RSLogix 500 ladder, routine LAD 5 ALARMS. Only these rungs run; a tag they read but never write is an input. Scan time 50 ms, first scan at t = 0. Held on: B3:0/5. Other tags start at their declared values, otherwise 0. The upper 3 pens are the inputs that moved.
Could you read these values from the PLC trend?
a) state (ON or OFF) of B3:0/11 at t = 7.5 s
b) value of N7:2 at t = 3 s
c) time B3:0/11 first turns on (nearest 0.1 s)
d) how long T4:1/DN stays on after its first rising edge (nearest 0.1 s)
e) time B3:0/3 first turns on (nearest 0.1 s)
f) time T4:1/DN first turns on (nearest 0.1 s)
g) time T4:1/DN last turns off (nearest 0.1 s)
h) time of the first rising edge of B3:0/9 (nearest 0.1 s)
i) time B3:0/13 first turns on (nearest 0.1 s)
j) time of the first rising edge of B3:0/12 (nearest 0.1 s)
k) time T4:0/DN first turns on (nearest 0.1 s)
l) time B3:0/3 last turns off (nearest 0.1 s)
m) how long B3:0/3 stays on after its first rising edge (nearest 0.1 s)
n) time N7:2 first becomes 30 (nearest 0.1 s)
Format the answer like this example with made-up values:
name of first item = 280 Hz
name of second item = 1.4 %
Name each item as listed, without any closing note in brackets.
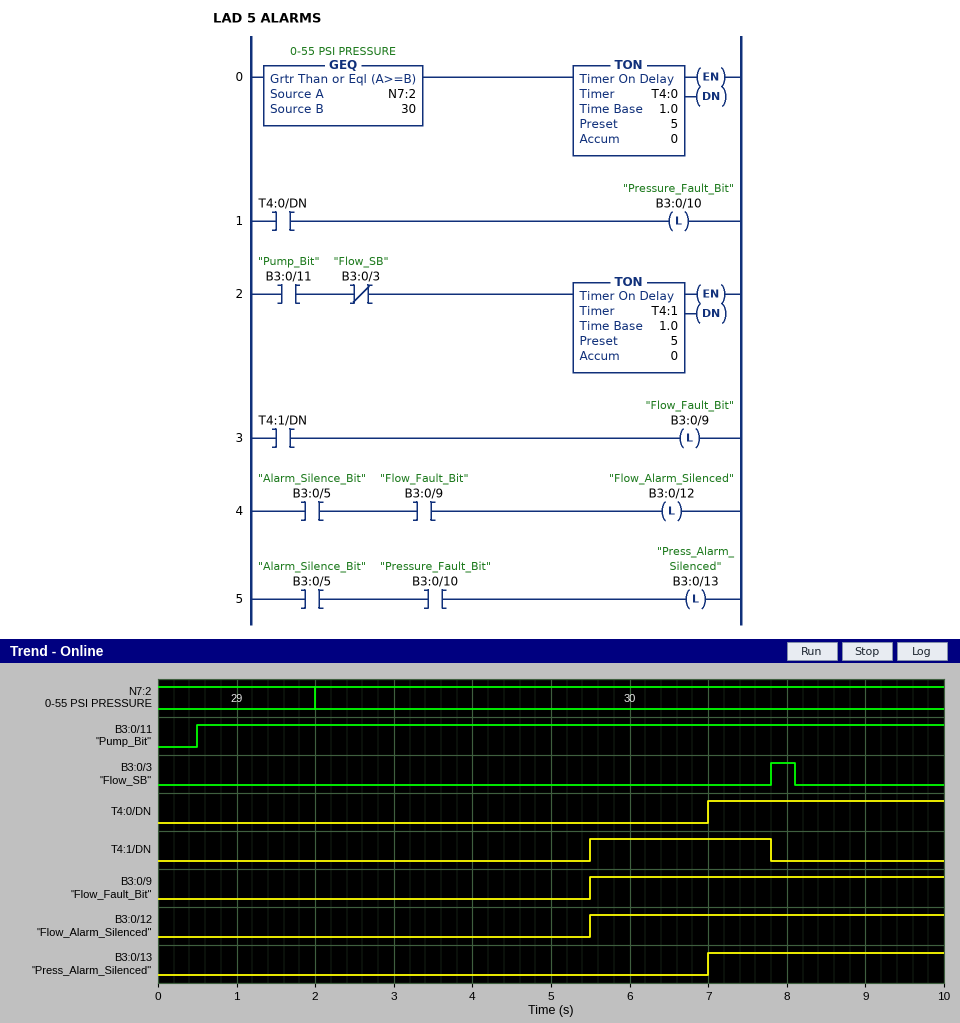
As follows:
state (ON or OFF) of B3:0/11 at t = 7.5 s = ON
value of N7:2 at t = 3 s = 30
time B3:0/11 first turns on = 0.5 s
how long T4:1/DN stays on after its first rising edge = 2.3 s
time B3:0/3 first turns on = 7.8 s
time T4:1/DN first turns on = 5.5 s
time T4:1/DN last turns off = 7.8 s
time of the first rising edge of B3:0/9 = 5.5 s
time B3:0/13 first turns on = 7.0 s
time of the first rising edge of B3:0/12 = 5.5 s
time T4:0/DN first turns on = 7.0 s
time B3:0/3 last turns off = 8.1 s
how long B3:0/3 stays on after its first rising edge = 0.3 s
time N7:2 first becomes 30 = 2.0 s
